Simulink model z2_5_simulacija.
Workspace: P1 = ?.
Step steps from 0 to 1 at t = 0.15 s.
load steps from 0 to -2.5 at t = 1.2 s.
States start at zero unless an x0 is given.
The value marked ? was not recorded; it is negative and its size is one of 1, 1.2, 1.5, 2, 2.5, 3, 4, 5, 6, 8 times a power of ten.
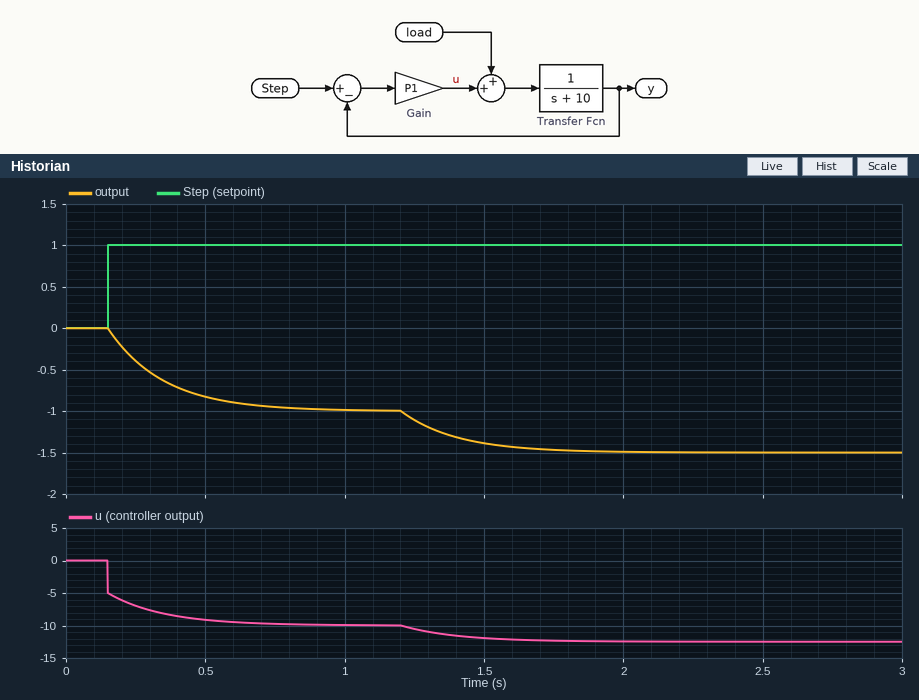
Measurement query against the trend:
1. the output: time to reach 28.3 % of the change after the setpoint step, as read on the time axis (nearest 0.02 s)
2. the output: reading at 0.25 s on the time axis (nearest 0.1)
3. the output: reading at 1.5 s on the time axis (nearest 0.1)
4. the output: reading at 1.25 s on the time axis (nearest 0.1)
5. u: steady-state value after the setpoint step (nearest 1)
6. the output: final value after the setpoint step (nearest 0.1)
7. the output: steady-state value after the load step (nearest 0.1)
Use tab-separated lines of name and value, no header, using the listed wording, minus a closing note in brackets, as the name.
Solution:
the output: time to reach 28.3 % of the change after the setpoint step, as read on the time axis	0.22 s
the output: reading at 0.25 s on the time axis	-0.4
the output: reading at 1.5 s on the time axis	-1.4
the output: reading at 1.25 s on the time axis	-1.1
u: steady-state value after the setpoint step	-10
the output: final value after the setpoint step	-1.0
the output: steady-state value after the load step	-1.5
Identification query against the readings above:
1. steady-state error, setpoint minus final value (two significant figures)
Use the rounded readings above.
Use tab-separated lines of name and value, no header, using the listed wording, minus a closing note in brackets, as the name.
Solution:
steady-state error, setpoint minus final value	2.0
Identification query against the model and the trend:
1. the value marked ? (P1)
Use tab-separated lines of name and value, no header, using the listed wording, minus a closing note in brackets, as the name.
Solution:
the value marked ?	-5
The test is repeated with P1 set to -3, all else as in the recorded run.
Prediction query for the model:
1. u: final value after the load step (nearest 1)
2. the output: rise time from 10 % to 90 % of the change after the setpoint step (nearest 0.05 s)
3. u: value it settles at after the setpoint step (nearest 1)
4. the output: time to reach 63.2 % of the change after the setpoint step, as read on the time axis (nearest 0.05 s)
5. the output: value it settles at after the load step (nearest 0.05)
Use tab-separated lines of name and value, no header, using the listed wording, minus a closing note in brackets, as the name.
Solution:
u: final value after the load step	-5
the output: rise time from 10 % to 90 % of the change after the setpoint step	0.30 s
u: value it settles at after the setpoint step	-4
the output: time to reach 63.2 % of the change after the setpoint step, as read on the time axis	0.30 s
the output: value it settles at after the load step	-0.80
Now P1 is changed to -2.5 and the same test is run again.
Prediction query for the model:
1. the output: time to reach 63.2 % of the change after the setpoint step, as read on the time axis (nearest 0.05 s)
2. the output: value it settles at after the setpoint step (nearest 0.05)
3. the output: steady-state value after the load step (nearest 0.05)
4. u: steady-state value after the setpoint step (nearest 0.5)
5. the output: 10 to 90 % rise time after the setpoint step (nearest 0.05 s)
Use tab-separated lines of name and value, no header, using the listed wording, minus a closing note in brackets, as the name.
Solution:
the output: time to reach 63.2 % of the change after the setpoint step, as read on the time axis	0.30 s
the output: value it settles at after the setpoint step	-0.35
the output: steady-state value after the load step	-0.65
u: steady-state value after the setpoint step	-3.5
the output: 10 to 90 % rise time after the setpoint step	0.30 s
